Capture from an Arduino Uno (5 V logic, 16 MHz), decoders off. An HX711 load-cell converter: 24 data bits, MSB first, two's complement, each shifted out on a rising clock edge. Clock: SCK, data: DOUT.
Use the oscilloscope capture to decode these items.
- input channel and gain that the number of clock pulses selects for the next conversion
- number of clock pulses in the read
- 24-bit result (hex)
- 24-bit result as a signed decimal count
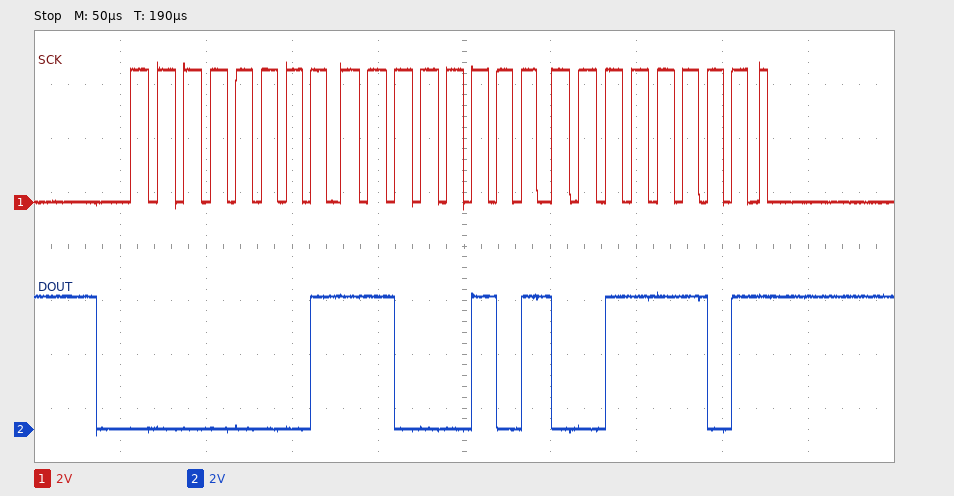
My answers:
channel A, gain 128
25
0x01C53D
116029
